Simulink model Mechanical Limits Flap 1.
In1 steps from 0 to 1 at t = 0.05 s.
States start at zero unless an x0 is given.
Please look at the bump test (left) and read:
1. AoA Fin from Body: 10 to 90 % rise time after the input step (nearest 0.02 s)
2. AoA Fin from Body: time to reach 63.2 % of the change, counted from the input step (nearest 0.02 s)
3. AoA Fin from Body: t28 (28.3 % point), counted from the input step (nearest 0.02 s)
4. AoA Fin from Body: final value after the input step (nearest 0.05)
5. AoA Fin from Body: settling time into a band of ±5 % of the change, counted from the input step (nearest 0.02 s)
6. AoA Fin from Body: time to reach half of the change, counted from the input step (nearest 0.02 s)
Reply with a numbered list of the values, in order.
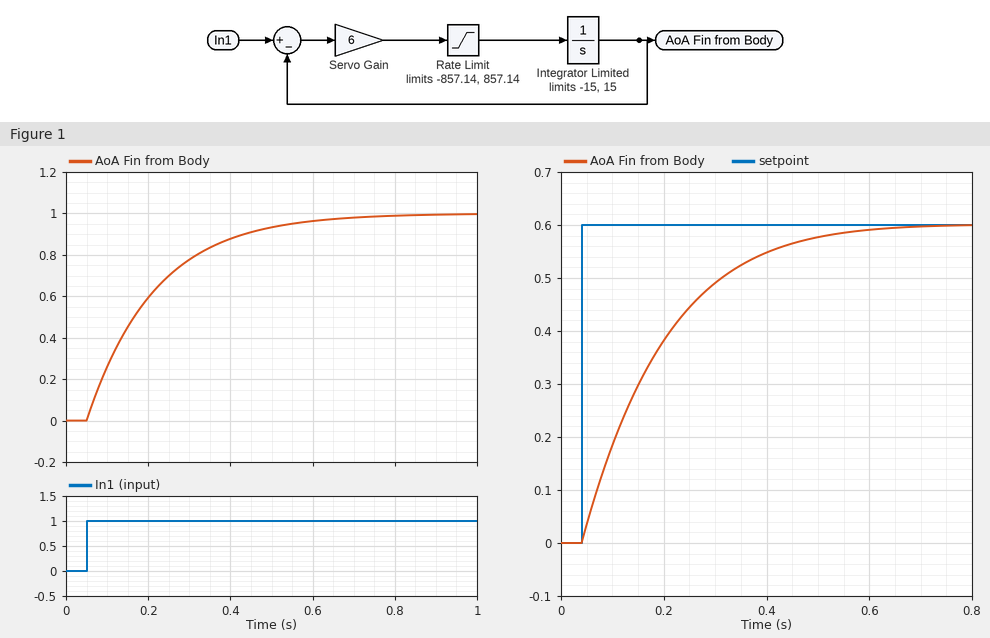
1. 0.36 s
2. 0.16 s
3. 0.06 s
4. 1.00
5. 0.50 s
6. 0.12 s
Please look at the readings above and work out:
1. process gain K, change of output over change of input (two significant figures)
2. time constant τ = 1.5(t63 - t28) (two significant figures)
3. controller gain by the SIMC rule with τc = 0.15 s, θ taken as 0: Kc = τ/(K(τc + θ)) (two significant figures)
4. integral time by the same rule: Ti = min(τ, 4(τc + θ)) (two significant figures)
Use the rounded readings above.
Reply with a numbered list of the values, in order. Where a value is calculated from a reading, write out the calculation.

1. (1 - 0) / 1 = 1.0
2. 1.5 × (0.16 - 0.06) = 0.15 s
3. 0.15 / (1 × (0.15 + 0)) = 1.0
4. min(0.15, 4 × (0.15 + 0)) = 0.15 s
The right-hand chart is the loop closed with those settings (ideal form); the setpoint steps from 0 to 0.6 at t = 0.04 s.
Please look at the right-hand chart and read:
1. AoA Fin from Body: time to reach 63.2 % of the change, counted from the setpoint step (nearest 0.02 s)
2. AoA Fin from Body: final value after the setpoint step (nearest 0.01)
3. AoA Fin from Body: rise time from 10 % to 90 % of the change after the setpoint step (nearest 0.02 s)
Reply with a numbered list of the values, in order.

1. 0.16 s
2. 0.60
3. 0.32 s
